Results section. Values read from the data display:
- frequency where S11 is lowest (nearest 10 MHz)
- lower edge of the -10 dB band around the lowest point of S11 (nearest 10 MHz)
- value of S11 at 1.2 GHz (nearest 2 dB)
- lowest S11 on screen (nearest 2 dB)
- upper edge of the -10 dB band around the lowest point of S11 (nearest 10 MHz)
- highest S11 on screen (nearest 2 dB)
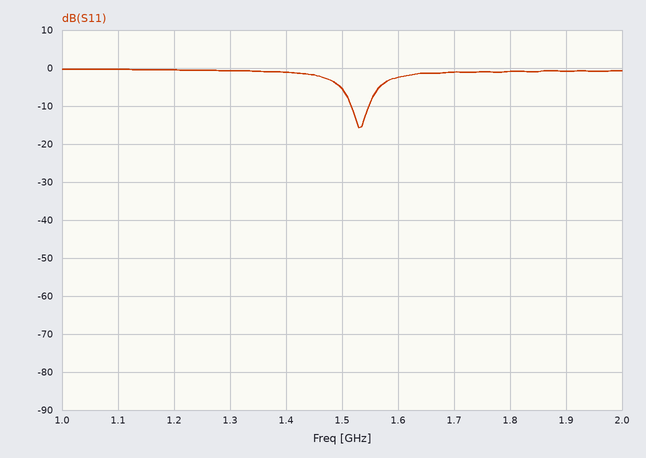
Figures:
1.53 GHz
1.52 GHz
0 dB
-16 dB
1.55 GHz
0 dB
